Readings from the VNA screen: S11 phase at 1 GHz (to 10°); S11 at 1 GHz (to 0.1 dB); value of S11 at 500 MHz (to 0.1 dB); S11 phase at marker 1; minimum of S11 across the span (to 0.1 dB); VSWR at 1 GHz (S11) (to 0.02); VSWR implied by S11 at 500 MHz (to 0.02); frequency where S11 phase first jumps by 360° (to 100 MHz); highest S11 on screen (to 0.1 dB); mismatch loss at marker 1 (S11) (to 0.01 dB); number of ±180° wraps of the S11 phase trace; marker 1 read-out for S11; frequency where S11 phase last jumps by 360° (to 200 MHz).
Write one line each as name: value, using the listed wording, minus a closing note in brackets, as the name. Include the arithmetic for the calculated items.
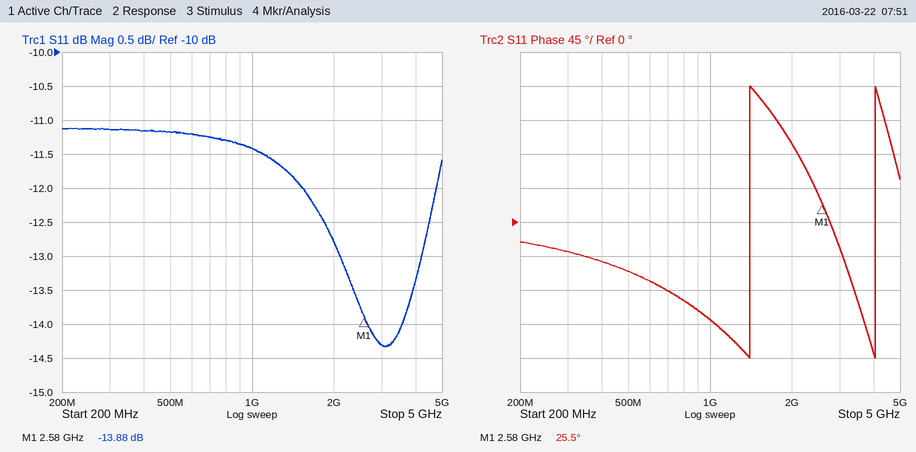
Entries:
S11 phase at 1 GHz: -130°
S11 at 1 GHz: -11.4 dB
value of S11 at 500 MHz: -11.2 dB
S11 phase at marker 1: 25.5°
minimum of S11 across the span: -14.3 dB
VSWR at 1 GHz (S11): |Γ| = 10^(-11.4/20) = 0.2692; VSWR = (1 + 0.2692)/(1 − 0.2692) ≈ 1.74
VSWR implied by S11 at 500 MHz: |Γ| = 10^(-11.2/20) = 0.2754; VSWR = (1 + 0.2754)/(1 − 0.2754) ≈ 1.76
frequency where S11 phase first jumps by 360°: 1.4 GHz
highest S11 on screen: -11.1 dB
mismatch loss at marker 1 (S11): −10 log10(1 − 10^(-13.88/10)) ≈ 0.18 dB
number of ±180° wraps of the S11 phase trace: 2
marker 1 read-out for S11: -13.88 dB
frequency where S11 phase last jumps by 360°: 4.0 GHz
